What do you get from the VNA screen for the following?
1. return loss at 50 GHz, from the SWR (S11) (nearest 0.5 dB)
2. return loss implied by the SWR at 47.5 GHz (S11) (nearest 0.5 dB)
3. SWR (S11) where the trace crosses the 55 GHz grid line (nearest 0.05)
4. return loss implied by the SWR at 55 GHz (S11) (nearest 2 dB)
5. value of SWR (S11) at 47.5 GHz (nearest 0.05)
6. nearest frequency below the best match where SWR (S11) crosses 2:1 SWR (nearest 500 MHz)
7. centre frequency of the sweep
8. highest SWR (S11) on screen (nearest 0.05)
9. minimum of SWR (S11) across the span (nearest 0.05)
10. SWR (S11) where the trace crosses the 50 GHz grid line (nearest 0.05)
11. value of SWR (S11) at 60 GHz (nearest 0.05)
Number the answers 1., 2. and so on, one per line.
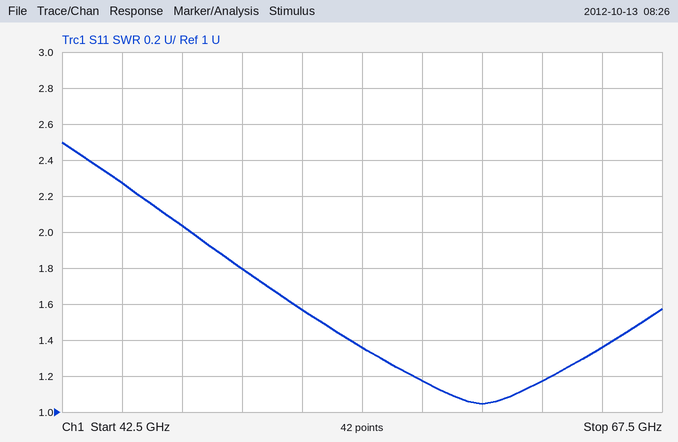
1. 11.0 dB
2. 9.5 dB
3. 1.35
4. 16 dB
5. 2.05
6. 48.0 GHz
7. 55 GHz
8. 2.50
9. 1.05
10. 1.80
11. 1.05
